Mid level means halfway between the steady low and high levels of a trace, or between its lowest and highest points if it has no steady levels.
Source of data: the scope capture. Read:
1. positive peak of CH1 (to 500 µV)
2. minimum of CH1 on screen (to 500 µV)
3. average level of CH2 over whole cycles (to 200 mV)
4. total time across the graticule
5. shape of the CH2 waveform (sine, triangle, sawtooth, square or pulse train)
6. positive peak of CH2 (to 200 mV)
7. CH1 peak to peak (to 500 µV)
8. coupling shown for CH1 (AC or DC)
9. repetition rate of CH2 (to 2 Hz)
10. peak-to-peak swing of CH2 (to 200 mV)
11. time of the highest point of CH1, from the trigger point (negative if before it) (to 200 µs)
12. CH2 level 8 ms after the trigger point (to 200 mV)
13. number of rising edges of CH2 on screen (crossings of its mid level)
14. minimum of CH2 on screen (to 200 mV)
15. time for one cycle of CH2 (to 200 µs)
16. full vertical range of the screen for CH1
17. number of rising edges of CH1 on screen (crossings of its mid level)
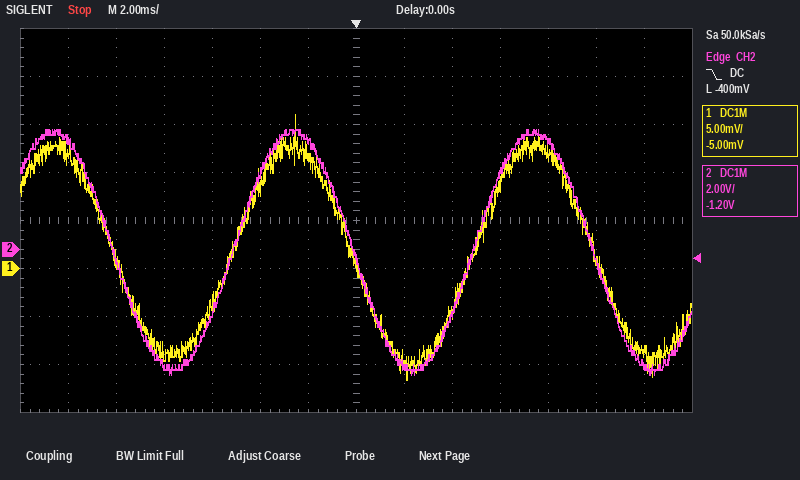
16.0 mV
-11.5 mV
0.0 V
28 ms
sine
5.0 V
27.5 mV
DC
100 Hz
10.2 V
-2.6 ms
4.6 V
2
-5.2 V
10.0 ms
40 mV
2
